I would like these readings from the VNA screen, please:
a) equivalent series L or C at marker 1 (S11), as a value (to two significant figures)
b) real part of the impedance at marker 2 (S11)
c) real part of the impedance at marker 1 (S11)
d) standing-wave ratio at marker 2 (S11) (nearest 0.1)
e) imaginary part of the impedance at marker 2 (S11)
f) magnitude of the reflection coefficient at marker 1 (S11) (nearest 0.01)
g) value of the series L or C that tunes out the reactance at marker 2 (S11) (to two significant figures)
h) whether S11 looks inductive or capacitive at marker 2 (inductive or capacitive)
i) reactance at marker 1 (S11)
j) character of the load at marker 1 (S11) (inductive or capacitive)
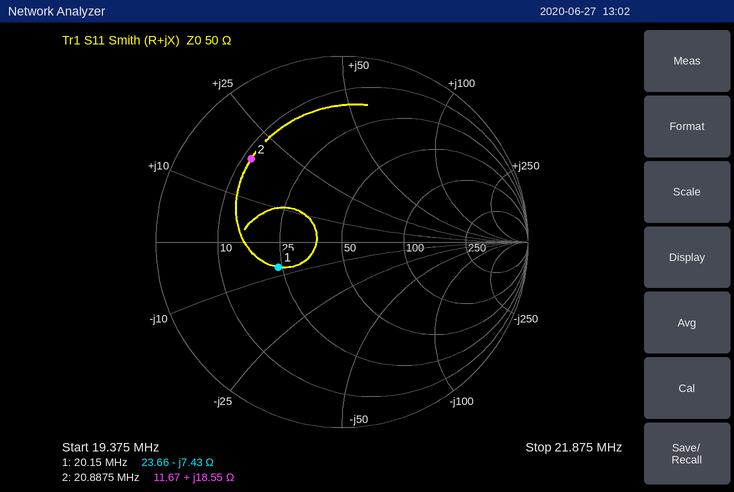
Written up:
1.1 nF
11.67 Ω
23.66 Ω
4.9
+18.55 Ω
0.37
410 pF
inductive
-7.43 Ω
capacitive
